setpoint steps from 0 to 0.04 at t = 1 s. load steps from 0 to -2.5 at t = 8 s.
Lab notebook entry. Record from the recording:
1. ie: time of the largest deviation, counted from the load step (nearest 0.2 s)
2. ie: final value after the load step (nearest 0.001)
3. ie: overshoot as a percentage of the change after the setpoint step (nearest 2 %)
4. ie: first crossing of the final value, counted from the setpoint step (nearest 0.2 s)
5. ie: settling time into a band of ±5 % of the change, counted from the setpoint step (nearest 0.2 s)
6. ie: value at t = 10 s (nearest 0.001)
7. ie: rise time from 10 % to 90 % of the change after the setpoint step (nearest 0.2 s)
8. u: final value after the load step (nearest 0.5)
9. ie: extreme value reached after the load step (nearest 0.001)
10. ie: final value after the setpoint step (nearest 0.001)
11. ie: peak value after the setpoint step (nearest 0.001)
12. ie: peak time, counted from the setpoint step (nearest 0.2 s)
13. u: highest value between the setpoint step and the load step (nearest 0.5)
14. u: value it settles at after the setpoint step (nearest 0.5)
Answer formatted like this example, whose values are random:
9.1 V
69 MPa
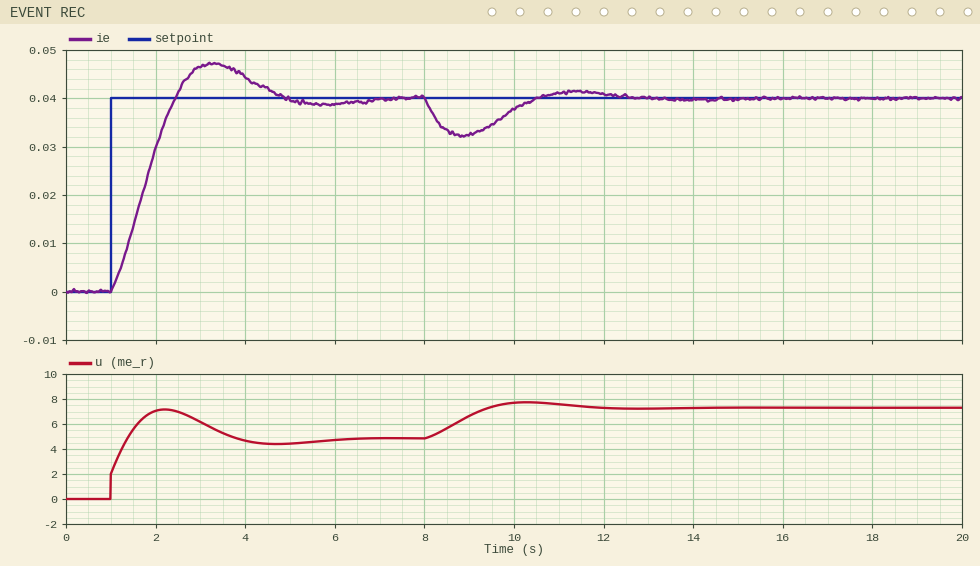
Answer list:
0.8 s
0.040
18 %
1.4 s
3.4 s
0.038
1.0 s
7.5
0.032
0.040
0.047
2.2 s
7.0
5.0
